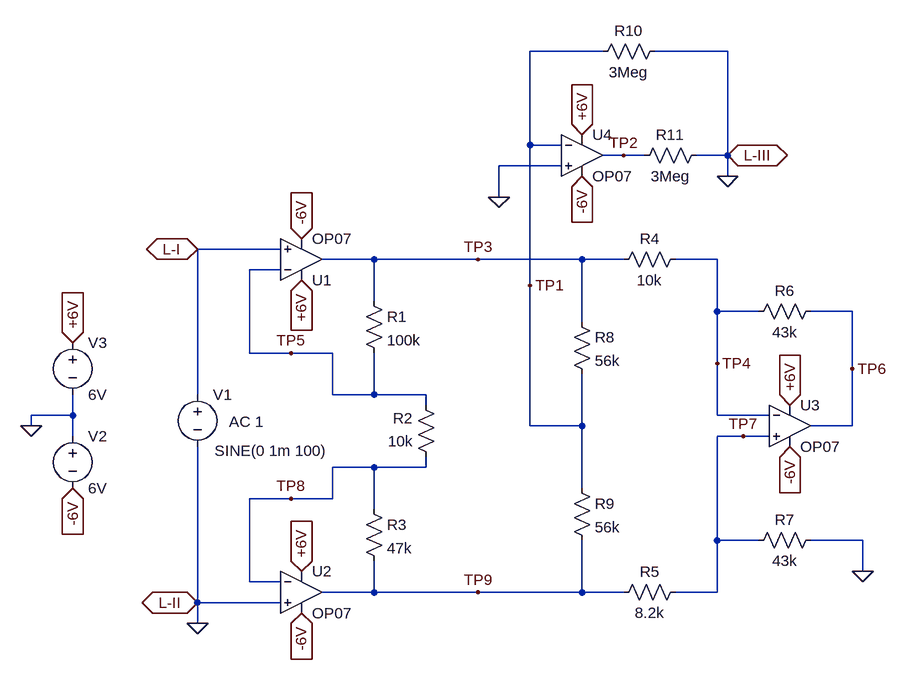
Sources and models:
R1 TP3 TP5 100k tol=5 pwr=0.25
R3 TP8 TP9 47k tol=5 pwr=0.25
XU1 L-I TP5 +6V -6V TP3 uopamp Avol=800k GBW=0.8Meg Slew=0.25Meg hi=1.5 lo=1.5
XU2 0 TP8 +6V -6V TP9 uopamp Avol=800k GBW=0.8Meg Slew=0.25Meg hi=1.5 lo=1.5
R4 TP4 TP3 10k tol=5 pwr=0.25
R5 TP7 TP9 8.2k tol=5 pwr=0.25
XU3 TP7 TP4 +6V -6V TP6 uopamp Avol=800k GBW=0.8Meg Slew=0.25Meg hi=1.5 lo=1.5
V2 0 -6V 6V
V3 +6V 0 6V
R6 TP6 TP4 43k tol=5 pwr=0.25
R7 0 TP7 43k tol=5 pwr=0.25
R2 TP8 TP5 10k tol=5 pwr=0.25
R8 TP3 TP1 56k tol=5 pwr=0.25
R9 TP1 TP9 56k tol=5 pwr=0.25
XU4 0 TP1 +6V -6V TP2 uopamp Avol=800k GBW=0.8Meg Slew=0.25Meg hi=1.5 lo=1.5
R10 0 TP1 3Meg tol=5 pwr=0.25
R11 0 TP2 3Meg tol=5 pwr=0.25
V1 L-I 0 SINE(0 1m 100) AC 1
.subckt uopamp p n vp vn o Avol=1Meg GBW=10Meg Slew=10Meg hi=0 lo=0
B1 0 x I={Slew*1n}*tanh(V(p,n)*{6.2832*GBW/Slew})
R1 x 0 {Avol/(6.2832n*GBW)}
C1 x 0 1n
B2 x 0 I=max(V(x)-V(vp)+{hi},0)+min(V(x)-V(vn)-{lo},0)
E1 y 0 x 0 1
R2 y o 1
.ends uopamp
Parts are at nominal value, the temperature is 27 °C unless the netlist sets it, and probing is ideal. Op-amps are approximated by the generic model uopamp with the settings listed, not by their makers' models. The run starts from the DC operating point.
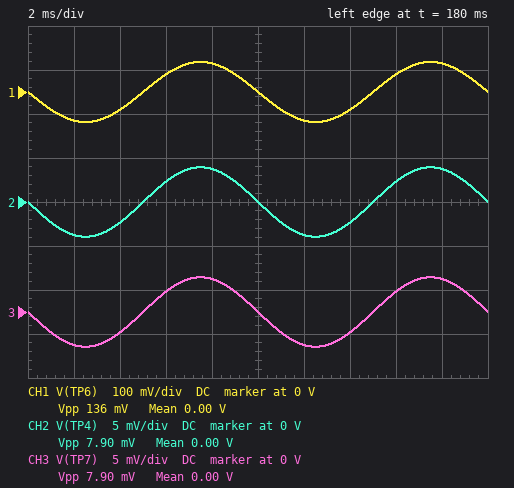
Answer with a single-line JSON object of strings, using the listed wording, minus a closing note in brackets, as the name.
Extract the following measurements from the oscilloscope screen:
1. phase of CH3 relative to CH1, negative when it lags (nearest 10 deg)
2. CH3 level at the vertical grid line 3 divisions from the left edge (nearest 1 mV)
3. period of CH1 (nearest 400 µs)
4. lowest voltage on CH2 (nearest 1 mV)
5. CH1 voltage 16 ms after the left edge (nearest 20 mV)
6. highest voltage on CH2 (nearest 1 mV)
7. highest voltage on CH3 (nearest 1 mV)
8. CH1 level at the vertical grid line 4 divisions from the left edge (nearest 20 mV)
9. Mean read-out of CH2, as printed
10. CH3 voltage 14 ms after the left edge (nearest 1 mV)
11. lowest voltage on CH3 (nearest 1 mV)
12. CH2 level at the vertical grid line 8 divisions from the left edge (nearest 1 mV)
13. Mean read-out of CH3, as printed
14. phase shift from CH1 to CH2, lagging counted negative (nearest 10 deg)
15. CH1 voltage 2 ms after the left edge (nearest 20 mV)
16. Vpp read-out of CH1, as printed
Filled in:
{"phase of CH3 relative to CH1, negative when it lags": "0 deg", "CH3 level at the vertical grid line 3 divisions from the left edge": "2 mV", "period of CH1": "10.0 ms", "lowest voltage on CH2": "-4 mV", "CH1 voltage 16 ms after the left edge": "40 mV", "highest voltage on CH2": "4 mV", "highest voltage on CH3": "4 mV", "CH1 level at the vertical grid line 4 divisions from the left edge": "60 mV", "Mean read-out of CH2, as printed": "0.00 V", "CH3 voltage 14 ms after the left edge": "-2 mV", "lowest voltage on CH3": "-4 mV", "CH2 level at the vertical grid line 8 divisions from the left edge": "2 mV", "Mean read-out of CH3, as printed": "0.00 V", "phase shift from CH1 to CH2, lagging counted negative": "0 deg", "CH1 voltage 2 ms after the left edge": "-60 mV", "Vpp read-out of CH1, as printed": "136 mV"}
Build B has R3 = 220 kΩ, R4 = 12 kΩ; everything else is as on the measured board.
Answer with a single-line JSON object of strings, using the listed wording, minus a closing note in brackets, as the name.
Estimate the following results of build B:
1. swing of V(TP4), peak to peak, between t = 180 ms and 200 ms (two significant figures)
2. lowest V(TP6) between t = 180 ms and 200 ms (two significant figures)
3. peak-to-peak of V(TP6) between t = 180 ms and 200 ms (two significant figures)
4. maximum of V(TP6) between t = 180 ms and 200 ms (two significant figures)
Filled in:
{"swing of V(TP4), peak to peak, between t = 180 ms and 200 ms": "37 mV", "lowest V(TP6) between t = 180 ms and 200 ms": "-120 mV", "peak-to-peak of V(TP6) between t = 180 ms and 200 ms": "250 mV", "maximum of V(TP6) between t = 180 ms and 200 ms": "120 mV"}
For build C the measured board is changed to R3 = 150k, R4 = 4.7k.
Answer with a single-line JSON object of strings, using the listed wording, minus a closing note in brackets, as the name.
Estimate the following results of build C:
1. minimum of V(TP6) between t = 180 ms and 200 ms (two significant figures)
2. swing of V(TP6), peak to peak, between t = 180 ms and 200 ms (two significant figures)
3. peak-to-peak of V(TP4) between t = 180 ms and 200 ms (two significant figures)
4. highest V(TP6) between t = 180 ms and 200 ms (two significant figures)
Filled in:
{"minimum of V(TP6) between t = 180 ms and 200 ms": "-230 mV", "swing of V(TP6), peak to peak, between t = 180 ms and 200 ms": "460 mV", "peak-to-peak of V(TP4) between t = 180 ms and 200 ms": "25 mV", "highest V(TP6) between t = 180 ms and 200 ms": "230 mV"}
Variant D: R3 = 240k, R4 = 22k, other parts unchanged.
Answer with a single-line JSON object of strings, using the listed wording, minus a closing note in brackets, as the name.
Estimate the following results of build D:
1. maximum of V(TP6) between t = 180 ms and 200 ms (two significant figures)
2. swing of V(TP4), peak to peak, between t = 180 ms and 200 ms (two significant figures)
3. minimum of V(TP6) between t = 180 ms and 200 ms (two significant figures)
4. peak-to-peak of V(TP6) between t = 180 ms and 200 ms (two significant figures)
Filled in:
{"maximum of V(TP6) between t = 180 ms and 200 ms": "81 mV", "swing of V(TP4), peak to peak, between t = 180 ms and 200 ms": "40 mV", "minimum of V(TP6) between t = 180 ms and 200 ms": "-81 mV", "peak-to-peak of V(TP6) between t = 180 ms and 200 ms": "160 mV"}
